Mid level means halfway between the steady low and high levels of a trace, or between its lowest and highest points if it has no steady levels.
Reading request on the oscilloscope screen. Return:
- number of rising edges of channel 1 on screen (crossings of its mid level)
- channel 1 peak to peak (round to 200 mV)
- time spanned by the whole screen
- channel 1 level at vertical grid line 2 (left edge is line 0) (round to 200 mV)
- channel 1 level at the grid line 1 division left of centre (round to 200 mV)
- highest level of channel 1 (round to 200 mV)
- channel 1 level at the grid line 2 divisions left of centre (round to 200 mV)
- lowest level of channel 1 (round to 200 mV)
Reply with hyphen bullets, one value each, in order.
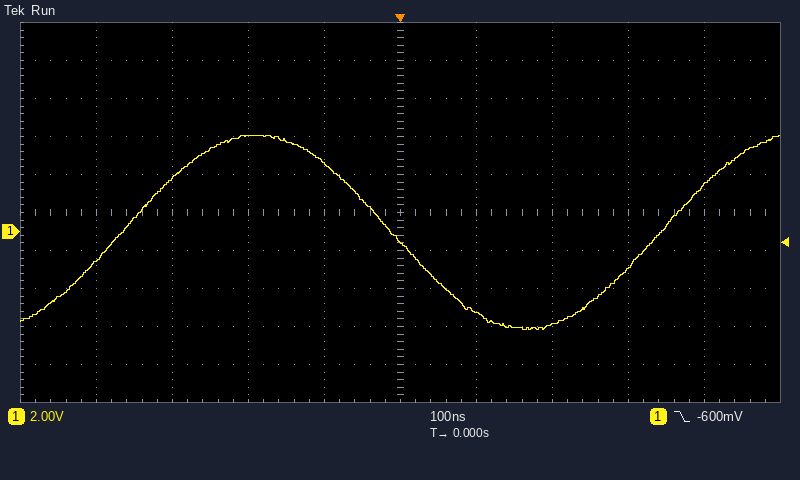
- 2
- 10.2 V
- 1 µs
- 2.8 V
- 3.6 V
- 5.0 V
- 5.0 V
- -5.2 V
